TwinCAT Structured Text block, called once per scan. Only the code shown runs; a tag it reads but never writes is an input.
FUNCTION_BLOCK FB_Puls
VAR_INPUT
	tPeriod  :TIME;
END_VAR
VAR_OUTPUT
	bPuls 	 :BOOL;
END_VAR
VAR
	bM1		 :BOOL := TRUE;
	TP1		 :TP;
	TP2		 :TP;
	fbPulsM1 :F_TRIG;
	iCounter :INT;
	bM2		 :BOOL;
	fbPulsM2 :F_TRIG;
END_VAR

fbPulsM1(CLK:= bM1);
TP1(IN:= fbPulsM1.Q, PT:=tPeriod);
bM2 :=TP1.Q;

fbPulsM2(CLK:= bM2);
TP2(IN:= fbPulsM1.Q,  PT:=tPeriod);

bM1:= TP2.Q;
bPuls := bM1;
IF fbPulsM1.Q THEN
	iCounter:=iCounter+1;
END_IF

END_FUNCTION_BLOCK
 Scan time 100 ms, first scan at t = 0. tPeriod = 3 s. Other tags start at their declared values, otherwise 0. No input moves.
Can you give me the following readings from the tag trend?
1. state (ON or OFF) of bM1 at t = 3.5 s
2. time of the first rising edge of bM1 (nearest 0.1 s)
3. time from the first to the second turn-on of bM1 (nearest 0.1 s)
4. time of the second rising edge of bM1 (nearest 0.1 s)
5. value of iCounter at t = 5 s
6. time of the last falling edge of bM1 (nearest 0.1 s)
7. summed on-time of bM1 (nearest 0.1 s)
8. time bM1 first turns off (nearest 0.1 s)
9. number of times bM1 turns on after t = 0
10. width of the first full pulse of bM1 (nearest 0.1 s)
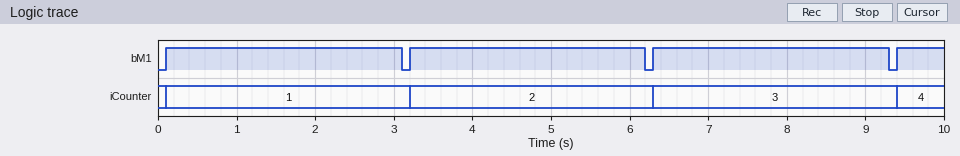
ON
0.1 s
3.1 s
3.2 s
2
9.3 s
9.6 s
3.1 s
4
3.0 s
